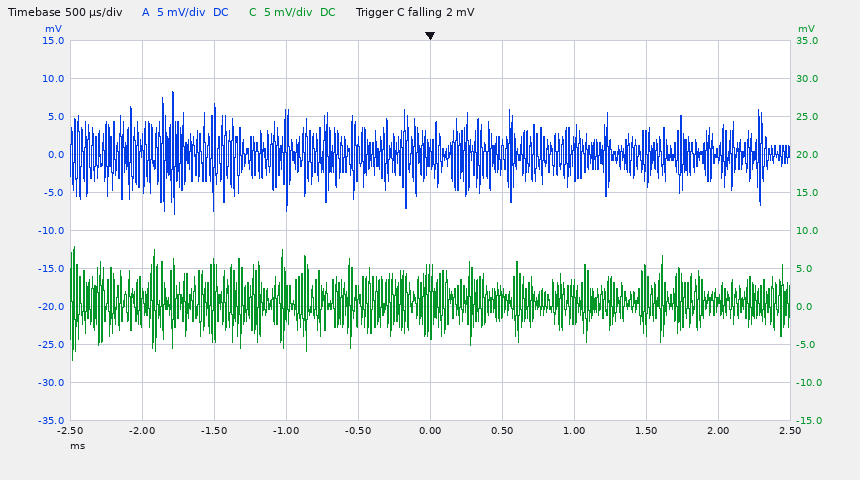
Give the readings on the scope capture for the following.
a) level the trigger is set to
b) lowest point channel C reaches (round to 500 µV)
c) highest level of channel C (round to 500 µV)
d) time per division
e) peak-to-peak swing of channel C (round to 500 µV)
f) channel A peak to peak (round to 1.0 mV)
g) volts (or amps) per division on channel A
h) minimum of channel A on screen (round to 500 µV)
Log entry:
2 mV
-7.0 mV
8.0 mV
500 µs
15.0 mV
16.0 mV
5 mV
-8.0 mV
